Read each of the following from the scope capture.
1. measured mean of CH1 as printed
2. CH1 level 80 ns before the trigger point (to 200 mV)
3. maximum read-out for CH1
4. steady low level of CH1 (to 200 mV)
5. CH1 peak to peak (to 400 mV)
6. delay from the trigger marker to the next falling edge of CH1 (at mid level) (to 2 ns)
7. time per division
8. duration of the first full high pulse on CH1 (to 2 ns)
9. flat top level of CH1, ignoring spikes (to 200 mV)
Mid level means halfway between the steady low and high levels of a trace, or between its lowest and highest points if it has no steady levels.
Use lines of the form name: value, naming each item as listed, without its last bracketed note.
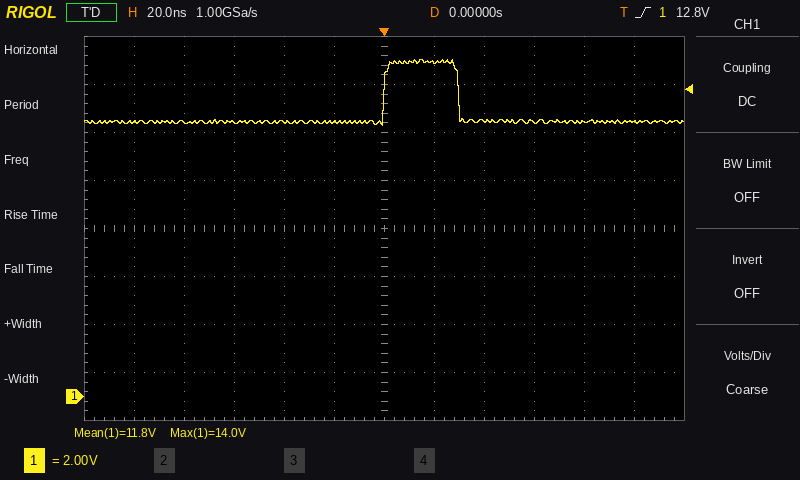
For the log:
measured mean of CH1 as printed: 11.8 V
CH1 level 80 ns before the trigger point: 11.4 V
maximum read-out for CH1: 14.0 V
steady low level of CH1: 11.4 V
CH1 peak to peak: 2.8 V
delay from the trigger marker to the next falling edge of CH1 (at mid level): 30 ns
time per division: 20 ns
duration of the first full high pulse on CH1: 30 ns
flat top level of CH1, ignoring spikes: 14.0 V
